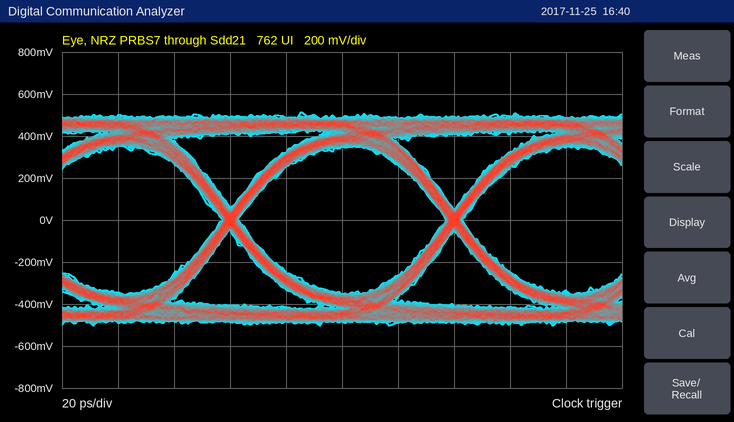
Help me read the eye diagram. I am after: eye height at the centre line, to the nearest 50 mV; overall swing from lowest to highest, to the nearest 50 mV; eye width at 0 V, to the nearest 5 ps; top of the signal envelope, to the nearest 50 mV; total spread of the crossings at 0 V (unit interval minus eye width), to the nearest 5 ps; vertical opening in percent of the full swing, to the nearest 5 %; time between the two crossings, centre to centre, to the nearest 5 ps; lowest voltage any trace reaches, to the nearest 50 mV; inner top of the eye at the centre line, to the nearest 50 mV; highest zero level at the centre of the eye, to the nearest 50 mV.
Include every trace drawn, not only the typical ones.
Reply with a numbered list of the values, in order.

1. 700 mV
2. 1.00 V
3. 75 ps
4. 500 mV
5. 5 ps
6. 70 %
7. 80 ps
8. -500 mV
9. 350 mV
10. -350 mV
